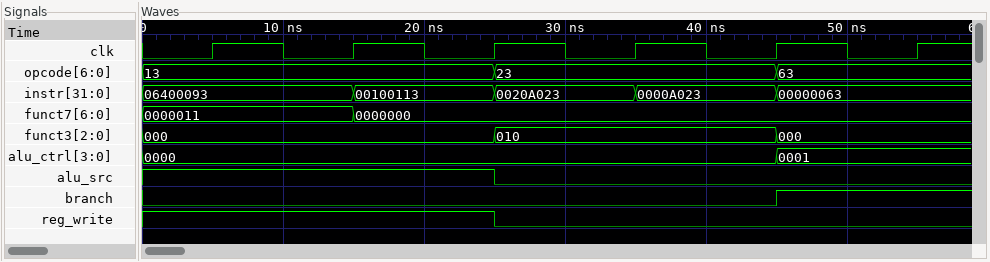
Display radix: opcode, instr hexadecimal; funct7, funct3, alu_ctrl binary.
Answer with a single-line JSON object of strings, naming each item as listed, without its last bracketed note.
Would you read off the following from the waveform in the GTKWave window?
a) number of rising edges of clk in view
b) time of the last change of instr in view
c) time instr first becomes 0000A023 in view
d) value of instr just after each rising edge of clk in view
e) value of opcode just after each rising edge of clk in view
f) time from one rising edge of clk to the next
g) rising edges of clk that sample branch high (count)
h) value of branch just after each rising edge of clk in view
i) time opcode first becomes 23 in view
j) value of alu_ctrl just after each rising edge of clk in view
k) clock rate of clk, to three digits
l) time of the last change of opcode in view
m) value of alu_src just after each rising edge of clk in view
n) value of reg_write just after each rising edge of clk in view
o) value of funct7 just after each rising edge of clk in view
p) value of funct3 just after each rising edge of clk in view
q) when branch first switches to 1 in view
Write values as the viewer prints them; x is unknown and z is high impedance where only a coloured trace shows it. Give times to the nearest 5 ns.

{"number of rising edges of clk in view": "6", "time of the last change of instr in view": "45 ns", "time instr first becomes 0000A023 in view": "35 ns", "value of instr just after each rising edge of clk in view": "06400093, 00100113, 0020A023, 0000A023, 00000063, 00000063", "value of opcode just after each rising edge of clk in view": "13, 13, 23, 23, 63, 63", "time from one rising edge of clk to the next": "10 ns", "rising edges of clk that sample branch high": "1", "value of branch just after each rising edge of clk in view": "0 0 0 0 1 1", "time opcode first becomes 23 in view": "25 ns", "value of alu_ctrl just after each rising edge of clk in view": "0000, 0000, 0000, 0000, 0001, 0001", "clock rate of clk, to three digits": "100 MHz", "time of the last change of opcode in view": "45 ns", "value of alu_src just after each rising edge of clk in view": "1 1 0 0 0 0", "value of reg_write just after each rising edge of clk in view": "1 1 0 0 0 0", "value of funct7 just after each rising edge of clk in view": "0000011, 0000000, 0000000, 0000000, 0000000, 0000000", "value of funct3 just after each rising edge of clk in view": "000, 000, 010, 010, 000, 000", "when branch first switches to 1 in view": "45 ns"}
